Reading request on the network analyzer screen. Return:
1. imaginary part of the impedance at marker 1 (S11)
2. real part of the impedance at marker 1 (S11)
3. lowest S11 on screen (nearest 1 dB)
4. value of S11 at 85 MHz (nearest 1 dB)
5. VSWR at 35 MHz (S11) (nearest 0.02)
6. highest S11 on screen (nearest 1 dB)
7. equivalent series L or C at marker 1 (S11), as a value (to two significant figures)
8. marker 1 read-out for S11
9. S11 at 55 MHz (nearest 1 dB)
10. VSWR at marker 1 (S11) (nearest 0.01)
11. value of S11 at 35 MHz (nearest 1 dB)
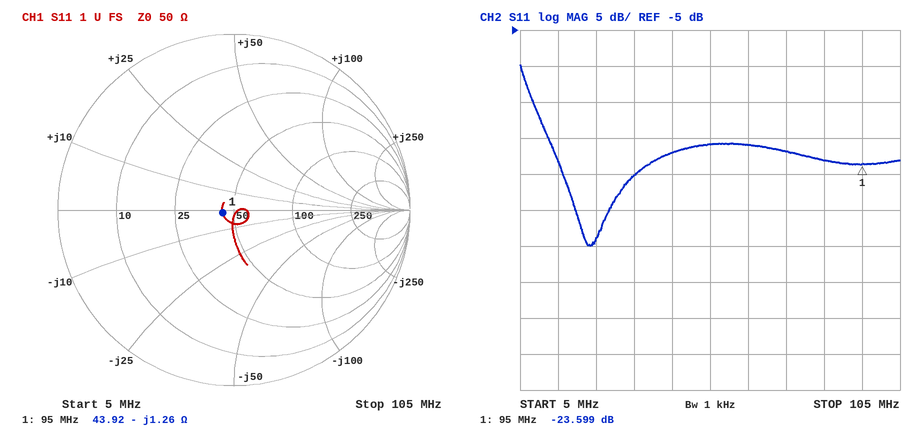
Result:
-1.26 Ω
43.92 Ω
-35 dB
-23 dB
1.12
-10 dB
1.3 nF
-23.599 dB
-21 dB
1.14
-25 dB
